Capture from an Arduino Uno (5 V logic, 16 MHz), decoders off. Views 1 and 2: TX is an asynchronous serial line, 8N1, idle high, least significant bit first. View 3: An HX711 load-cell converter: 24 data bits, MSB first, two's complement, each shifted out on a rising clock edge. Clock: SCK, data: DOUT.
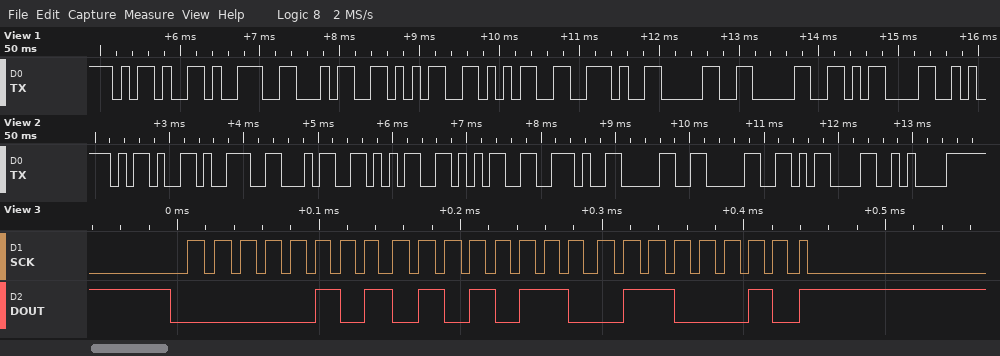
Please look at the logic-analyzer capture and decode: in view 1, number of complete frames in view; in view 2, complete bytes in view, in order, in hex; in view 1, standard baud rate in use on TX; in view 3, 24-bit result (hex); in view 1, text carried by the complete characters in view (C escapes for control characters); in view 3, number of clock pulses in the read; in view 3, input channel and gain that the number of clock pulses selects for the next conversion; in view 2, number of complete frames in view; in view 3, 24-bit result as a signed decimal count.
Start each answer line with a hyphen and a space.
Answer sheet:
- 9
- 2D 39 34 35 35 2E 30 30 0D 0A
- 9600 baud
- 0x055662
- "-9455.00\r"
- 25
- channel A, gain 128
- 10
- 349794
